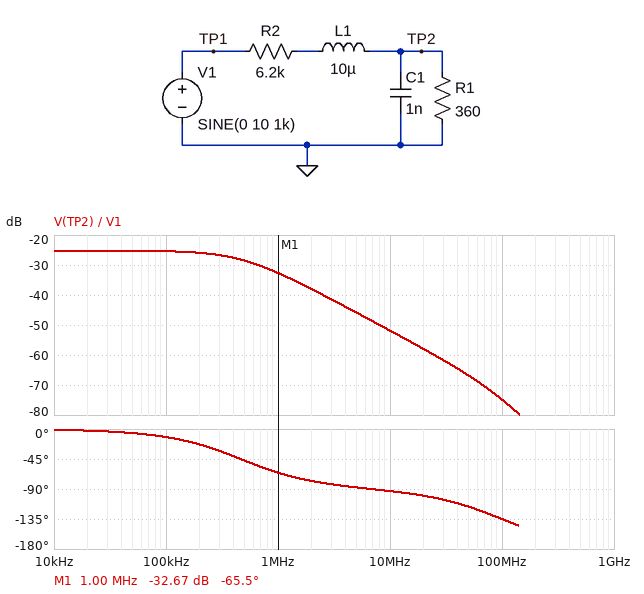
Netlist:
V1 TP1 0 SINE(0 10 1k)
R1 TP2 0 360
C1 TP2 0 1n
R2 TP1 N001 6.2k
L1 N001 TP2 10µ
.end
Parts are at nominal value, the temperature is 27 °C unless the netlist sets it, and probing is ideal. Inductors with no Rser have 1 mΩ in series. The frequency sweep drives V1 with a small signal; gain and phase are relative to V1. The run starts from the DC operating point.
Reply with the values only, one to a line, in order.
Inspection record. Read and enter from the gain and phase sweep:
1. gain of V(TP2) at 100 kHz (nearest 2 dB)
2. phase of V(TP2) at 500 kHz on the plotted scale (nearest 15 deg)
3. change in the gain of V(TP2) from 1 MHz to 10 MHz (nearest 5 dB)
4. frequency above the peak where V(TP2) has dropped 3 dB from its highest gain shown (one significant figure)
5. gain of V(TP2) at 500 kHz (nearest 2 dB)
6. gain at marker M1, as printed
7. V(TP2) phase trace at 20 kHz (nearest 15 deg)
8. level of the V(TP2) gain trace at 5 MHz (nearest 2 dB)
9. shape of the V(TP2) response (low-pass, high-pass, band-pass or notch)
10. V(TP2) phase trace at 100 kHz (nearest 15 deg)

-26 dB
-45 deg
-20 dB
500 kHz
-28 dB
-32.67 dB
0 deg
-46 dB
low-pass
-15 deg
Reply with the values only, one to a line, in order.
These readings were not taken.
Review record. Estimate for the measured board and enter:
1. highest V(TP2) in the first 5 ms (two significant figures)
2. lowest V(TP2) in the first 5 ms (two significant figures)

550 mV
-550 mV
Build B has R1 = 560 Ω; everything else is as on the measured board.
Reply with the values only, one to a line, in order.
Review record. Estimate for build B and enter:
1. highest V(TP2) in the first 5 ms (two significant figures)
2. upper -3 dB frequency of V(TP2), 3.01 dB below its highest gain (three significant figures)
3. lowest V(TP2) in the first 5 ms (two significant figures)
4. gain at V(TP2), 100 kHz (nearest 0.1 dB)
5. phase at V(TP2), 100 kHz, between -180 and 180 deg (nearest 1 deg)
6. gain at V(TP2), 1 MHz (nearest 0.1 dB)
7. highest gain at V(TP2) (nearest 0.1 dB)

830 mV
310 kHz
-830 mV
-22.1 dB
-18 deg
-32.2 dB
-21.6 dB
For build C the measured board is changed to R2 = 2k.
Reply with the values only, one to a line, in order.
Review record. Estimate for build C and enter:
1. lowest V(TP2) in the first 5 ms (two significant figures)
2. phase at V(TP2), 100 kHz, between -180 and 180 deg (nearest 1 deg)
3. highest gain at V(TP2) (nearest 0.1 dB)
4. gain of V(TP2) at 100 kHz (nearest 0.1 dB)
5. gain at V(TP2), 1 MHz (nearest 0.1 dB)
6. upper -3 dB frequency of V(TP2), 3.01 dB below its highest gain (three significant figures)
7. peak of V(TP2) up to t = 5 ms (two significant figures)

-1.5 V
-11 deg
-16.3 dB
-16.5 dB
-23.0 dB
523 kHz
1.5 V
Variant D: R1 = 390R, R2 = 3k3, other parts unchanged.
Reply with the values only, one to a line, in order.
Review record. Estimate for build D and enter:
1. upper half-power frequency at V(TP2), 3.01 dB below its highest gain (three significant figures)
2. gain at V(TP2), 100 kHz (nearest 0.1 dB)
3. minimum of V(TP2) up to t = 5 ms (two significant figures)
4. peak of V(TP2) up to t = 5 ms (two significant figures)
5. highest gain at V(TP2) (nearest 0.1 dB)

457 kHz
-19.7 dB
-1.1 V
1.1 V
-19.5 dB
